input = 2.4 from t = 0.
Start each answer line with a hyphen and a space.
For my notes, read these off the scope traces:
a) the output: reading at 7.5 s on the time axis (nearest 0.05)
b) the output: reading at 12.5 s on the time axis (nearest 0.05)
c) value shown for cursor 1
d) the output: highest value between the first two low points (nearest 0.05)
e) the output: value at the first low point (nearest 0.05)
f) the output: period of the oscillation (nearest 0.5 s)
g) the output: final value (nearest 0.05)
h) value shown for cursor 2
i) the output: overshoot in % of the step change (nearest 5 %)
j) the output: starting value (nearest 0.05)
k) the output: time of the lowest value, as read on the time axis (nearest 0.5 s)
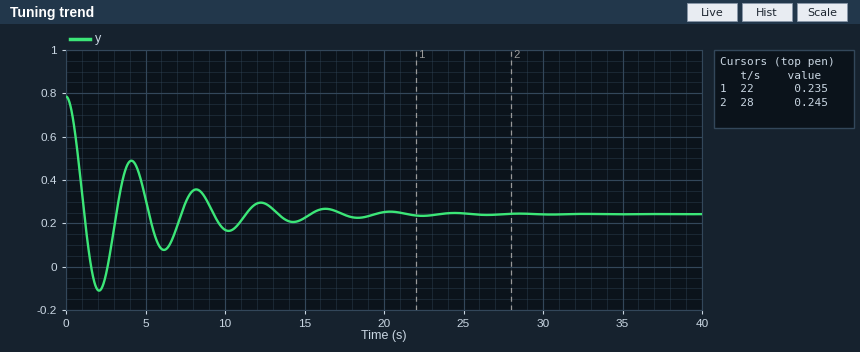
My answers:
- 0.30
- 0.30
- 0.235
- 0.50
- -0.10
- 4.0 s
- 0.25
- 0.245
- 65 %
- 0.80
- 2.0 s
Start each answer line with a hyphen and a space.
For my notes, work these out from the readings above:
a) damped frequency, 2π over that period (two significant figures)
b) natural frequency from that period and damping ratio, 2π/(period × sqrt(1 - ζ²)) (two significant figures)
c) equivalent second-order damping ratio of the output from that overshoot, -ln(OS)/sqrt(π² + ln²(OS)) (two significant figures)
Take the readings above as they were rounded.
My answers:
- 1.6 rad/s
- 1.6 rad/s
- 0.14
